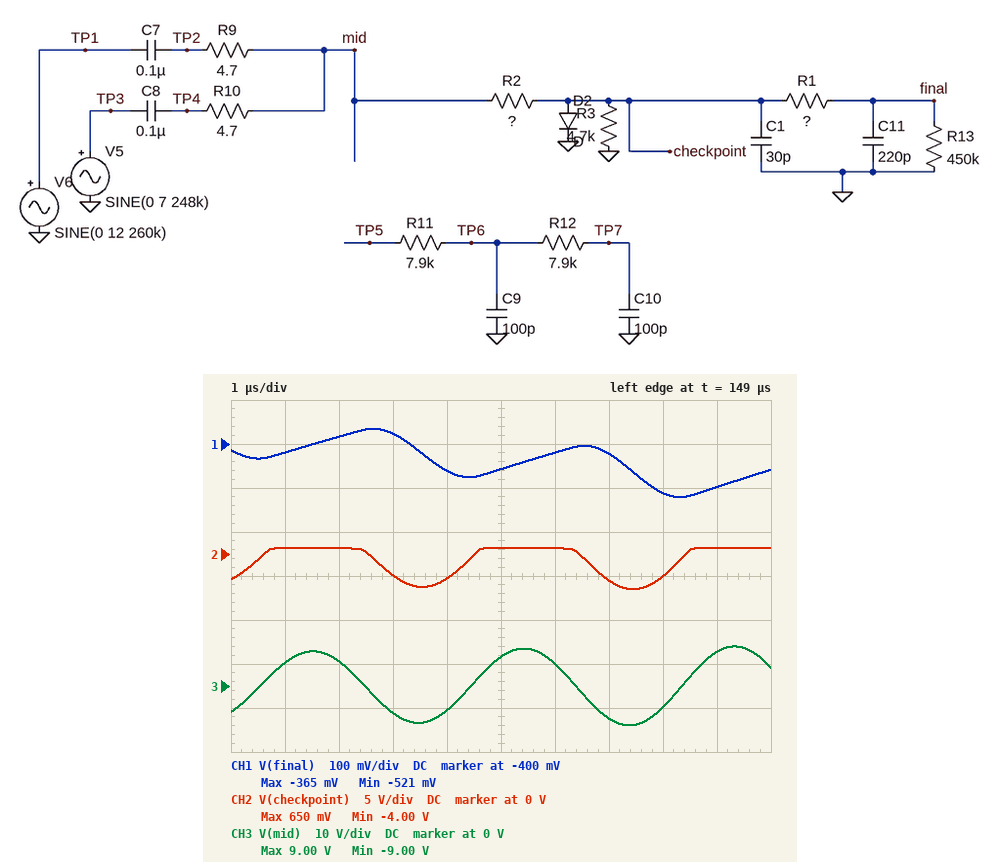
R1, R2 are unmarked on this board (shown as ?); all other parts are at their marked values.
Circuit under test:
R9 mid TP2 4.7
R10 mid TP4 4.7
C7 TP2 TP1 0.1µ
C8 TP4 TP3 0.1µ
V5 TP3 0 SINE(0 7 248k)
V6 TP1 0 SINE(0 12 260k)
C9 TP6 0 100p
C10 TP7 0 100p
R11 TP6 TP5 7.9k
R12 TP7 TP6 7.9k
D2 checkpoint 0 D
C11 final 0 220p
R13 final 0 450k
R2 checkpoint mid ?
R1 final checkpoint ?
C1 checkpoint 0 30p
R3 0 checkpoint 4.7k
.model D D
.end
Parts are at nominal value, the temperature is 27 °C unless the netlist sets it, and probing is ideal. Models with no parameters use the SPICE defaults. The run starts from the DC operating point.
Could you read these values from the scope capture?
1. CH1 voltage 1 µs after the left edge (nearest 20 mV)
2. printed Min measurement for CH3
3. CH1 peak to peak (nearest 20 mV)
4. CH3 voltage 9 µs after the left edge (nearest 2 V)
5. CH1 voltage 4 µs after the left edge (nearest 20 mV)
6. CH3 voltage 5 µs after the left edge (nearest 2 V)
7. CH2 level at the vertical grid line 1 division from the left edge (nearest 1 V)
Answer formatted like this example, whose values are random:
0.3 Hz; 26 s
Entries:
-420 mV; -9.00 V; 160 mV; 8 V; -460 mV; 6 V; 1 V
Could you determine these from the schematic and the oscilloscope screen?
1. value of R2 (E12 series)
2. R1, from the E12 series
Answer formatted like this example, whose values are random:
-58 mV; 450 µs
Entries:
5.6 kΩ; 150 kΩ
